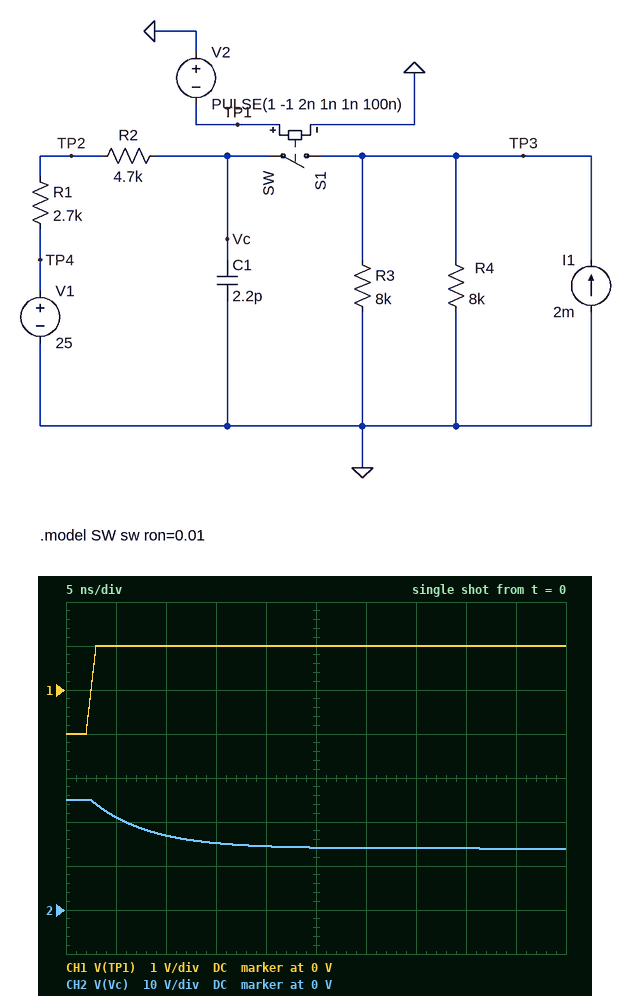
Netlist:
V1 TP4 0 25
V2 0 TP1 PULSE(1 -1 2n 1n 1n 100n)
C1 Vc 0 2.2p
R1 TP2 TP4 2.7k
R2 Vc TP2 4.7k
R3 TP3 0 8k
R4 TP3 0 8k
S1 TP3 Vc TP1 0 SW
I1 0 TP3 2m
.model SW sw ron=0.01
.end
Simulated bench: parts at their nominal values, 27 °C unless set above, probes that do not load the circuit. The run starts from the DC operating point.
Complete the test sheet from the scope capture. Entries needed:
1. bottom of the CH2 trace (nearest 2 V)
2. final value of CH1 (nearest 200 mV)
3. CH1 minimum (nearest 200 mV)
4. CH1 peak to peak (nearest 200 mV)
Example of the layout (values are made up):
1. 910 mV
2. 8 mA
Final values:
1. 14 V
2. 1.0 V
3. -1.0 V
4. 2.0 V
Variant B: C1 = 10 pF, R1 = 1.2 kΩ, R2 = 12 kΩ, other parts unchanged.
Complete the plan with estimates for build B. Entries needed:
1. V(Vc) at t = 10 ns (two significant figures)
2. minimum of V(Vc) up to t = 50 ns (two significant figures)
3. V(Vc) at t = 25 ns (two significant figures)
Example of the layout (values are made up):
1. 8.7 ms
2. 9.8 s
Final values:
1. 22 V
2. 15 V
3. 18 V
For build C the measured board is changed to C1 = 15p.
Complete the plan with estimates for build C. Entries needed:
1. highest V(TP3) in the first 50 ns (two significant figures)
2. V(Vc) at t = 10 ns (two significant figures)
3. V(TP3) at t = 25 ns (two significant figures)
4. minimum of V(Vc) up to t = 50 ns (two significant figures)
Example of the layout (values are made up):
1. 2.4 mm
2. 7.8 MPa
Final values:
1. 25 V
2. 23 V
3. 20 V
4. 17 V
